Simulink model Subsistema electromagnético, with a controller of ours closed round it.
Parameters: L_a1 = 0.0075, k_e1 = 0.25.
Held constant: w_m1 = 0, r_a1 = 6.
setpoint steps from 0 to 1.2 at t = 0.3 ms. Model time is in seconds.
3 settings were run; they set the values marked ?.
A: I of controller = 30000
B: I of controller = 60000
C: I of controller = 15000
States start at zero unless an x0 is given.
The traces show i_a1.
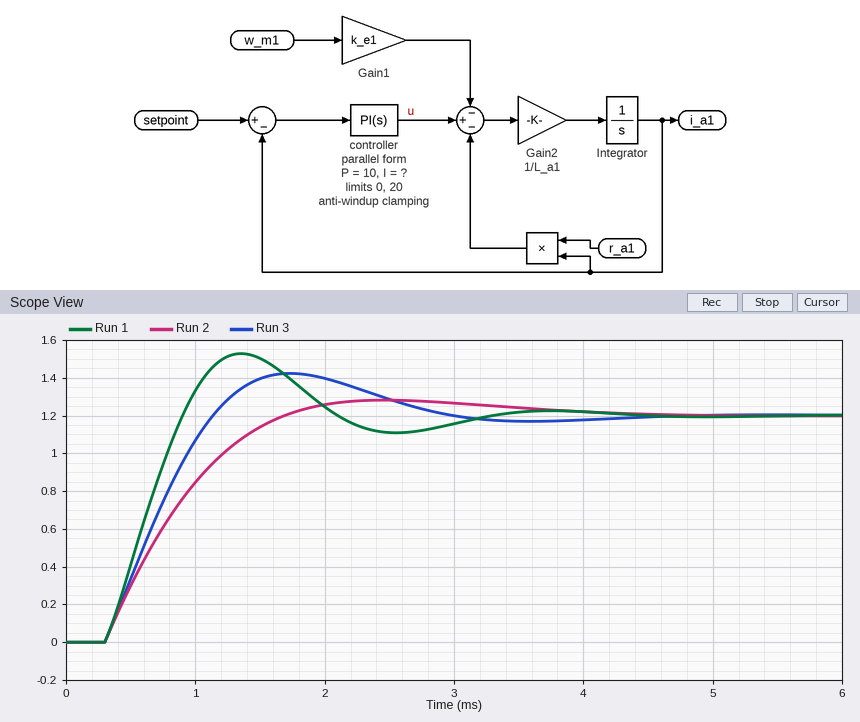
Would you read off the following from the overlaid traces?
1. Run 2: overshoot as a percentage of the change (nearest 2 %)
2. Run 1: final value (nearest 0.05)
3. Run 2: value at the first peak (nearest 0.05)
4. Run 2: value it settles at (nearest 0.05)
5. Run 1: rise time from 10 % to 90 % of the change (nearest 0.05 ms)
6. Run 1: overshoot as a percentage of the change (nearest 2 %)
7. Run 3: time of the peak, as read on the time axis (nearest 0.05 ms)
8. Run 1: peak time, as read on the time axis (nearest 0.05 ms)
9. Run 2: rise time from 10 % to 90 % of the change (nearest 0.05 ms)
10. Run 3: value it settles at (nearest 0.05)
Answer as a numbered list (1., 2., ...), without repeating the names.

1. 6 %
2. 1.20
3. 1.30
4. 1.20
5. 0.45 ms
6. 28 %
7. 1.75 ms
8. 1.35 ms
9. 1.00 ms
10. 1.20
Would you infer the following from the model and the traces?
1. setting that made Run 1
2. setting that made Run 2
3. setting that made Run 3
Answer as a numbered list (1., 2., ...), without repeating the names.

1. B
2. C
3. A
